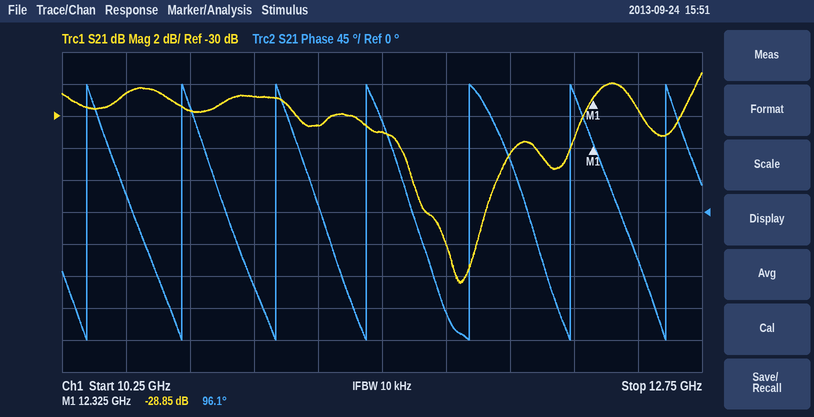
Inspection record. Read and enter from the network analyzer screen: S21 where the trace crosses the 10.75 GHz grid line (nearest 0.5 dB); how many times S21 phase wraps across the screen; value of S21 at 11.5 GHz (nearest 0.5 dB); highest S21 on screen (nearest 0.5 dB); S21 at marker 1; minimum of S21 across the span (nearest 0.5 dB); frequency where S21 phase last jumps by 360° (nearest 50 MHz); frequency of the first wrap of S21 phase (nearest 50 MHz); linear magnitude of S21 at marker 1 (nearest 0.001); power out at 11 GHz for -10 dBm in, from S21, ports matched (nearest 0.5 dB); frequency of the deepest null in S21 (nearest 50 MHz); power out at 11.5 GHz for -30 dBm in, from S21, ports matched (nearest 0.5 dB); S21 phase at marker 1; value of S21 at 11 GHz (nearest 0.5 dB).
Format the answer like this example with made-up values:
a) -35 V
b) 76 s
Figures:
a) -29.5 dB
b) 7
c) -31.0 dB
d) -27.5 dB
e) -28.85 dB
f) -40.5 dB
g) 12.60 GHz
h) 10.35 GHz
i) 0.036
j) -39.0 dBm
k) 11.80 GHz
l) -61.0 dBm
m) 96.1°
n) -29.0 dB
